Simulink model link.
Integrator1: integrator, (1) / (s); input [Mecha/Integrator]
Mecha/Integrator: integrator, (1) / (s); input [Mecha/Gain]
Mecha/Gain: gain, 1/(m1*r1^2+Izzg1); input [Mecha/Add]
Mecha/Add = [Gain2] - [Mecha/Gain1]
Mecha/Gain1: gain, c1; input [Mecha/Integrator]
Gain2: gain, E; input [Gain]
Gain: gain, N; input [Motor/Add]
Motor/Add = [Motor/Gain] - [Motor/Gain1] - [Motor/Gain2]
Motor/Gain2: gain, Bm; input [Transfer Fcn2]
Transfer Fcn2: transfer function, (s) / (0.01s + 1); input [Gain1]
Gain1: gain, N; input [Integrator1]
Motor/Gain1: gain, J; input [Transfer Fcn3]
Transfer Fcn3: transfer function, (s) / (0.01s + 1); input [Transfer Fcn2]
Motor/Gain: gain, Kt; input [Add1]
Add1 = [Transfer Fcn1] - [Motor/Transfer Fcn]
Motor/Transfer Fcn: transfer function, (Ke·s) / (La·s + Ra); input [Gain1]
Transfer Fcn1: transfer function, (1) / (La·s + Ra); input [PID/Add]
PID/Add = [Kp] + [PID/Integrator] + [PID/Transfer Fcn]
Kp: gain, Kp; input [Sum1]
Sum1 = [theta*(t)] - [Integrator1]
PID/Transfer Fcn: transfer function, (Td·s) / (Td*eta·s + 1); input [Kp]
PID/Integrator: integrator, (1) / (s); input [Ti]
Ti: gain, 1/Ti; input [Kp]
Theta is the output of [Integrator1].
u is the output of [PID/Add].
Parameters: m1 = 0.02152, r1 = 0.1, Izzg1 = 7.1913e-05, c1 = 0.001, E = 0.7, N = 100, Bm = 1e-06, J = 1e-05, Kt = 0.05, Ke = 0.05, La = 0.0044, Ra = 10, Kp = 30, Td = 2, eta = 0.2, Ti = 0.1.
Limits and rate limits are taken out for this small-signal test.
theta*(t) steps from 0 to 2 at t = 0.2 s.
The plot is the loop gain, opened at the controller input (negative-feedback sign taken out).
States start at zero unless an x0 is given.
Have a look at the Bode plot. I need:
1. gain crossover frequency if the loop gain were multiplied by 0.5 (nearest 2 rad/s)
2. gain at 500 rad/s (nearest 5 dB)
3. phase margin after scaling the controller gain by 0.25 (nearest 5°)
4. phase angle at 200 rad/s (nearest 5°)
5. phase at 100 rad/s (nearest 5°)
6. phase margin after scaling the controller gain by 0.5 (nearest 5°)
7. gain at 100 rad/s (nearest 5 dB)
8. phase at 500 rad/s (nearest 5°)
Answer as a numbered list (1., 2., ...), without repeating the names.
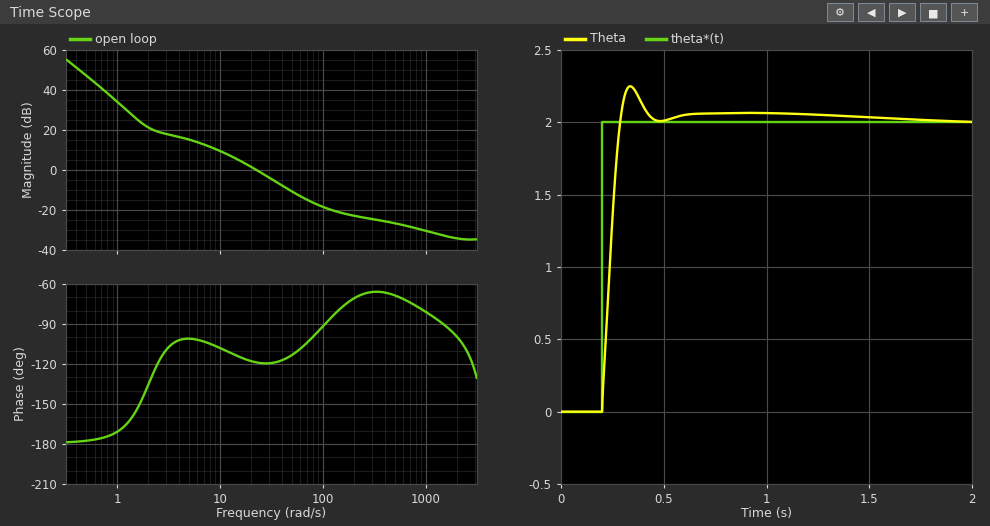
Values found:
1. 14 rad/s
2. -25 dB
3. 75°
4. -70°
5. -90°
6. 65°
7. -20 dB
8. -70°
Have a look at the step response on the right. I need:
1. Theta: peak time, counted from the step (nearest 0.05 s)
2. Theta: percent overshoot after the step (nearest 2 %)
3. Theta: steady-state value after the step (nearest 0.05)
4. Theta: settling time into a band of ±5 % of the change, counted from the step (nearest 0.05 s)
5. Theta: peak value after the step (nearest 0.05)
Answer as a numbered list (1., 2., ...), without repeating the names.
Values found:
1. 0.15 s
2. 12 %
3. 2.00
4. 0.20 s
5. 2.25
